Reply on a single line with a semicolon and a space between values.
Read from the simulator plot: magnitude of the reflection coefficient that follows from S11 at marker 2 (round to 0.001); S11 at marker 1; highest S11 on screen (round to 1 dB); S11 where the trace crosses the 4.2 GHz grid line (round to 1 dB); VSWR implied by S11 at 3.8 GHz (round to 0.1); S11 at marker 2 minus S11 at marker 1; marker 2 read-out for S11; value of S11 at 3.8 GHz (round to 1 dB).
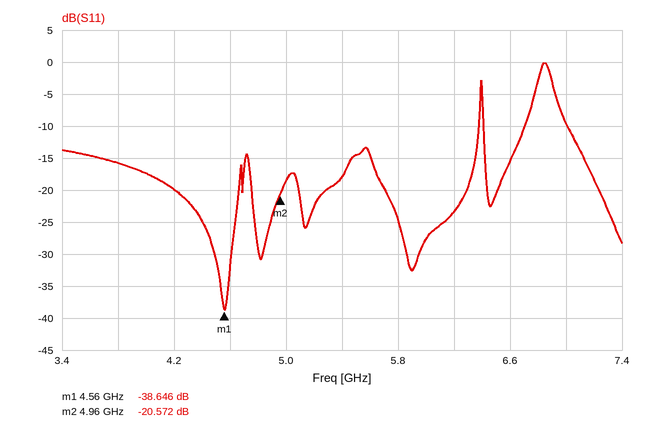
0.094; -38.646 dB; 0 dB; -20 dB; 1.4; 18.074 dB; -20.572 dB; -16 dB
